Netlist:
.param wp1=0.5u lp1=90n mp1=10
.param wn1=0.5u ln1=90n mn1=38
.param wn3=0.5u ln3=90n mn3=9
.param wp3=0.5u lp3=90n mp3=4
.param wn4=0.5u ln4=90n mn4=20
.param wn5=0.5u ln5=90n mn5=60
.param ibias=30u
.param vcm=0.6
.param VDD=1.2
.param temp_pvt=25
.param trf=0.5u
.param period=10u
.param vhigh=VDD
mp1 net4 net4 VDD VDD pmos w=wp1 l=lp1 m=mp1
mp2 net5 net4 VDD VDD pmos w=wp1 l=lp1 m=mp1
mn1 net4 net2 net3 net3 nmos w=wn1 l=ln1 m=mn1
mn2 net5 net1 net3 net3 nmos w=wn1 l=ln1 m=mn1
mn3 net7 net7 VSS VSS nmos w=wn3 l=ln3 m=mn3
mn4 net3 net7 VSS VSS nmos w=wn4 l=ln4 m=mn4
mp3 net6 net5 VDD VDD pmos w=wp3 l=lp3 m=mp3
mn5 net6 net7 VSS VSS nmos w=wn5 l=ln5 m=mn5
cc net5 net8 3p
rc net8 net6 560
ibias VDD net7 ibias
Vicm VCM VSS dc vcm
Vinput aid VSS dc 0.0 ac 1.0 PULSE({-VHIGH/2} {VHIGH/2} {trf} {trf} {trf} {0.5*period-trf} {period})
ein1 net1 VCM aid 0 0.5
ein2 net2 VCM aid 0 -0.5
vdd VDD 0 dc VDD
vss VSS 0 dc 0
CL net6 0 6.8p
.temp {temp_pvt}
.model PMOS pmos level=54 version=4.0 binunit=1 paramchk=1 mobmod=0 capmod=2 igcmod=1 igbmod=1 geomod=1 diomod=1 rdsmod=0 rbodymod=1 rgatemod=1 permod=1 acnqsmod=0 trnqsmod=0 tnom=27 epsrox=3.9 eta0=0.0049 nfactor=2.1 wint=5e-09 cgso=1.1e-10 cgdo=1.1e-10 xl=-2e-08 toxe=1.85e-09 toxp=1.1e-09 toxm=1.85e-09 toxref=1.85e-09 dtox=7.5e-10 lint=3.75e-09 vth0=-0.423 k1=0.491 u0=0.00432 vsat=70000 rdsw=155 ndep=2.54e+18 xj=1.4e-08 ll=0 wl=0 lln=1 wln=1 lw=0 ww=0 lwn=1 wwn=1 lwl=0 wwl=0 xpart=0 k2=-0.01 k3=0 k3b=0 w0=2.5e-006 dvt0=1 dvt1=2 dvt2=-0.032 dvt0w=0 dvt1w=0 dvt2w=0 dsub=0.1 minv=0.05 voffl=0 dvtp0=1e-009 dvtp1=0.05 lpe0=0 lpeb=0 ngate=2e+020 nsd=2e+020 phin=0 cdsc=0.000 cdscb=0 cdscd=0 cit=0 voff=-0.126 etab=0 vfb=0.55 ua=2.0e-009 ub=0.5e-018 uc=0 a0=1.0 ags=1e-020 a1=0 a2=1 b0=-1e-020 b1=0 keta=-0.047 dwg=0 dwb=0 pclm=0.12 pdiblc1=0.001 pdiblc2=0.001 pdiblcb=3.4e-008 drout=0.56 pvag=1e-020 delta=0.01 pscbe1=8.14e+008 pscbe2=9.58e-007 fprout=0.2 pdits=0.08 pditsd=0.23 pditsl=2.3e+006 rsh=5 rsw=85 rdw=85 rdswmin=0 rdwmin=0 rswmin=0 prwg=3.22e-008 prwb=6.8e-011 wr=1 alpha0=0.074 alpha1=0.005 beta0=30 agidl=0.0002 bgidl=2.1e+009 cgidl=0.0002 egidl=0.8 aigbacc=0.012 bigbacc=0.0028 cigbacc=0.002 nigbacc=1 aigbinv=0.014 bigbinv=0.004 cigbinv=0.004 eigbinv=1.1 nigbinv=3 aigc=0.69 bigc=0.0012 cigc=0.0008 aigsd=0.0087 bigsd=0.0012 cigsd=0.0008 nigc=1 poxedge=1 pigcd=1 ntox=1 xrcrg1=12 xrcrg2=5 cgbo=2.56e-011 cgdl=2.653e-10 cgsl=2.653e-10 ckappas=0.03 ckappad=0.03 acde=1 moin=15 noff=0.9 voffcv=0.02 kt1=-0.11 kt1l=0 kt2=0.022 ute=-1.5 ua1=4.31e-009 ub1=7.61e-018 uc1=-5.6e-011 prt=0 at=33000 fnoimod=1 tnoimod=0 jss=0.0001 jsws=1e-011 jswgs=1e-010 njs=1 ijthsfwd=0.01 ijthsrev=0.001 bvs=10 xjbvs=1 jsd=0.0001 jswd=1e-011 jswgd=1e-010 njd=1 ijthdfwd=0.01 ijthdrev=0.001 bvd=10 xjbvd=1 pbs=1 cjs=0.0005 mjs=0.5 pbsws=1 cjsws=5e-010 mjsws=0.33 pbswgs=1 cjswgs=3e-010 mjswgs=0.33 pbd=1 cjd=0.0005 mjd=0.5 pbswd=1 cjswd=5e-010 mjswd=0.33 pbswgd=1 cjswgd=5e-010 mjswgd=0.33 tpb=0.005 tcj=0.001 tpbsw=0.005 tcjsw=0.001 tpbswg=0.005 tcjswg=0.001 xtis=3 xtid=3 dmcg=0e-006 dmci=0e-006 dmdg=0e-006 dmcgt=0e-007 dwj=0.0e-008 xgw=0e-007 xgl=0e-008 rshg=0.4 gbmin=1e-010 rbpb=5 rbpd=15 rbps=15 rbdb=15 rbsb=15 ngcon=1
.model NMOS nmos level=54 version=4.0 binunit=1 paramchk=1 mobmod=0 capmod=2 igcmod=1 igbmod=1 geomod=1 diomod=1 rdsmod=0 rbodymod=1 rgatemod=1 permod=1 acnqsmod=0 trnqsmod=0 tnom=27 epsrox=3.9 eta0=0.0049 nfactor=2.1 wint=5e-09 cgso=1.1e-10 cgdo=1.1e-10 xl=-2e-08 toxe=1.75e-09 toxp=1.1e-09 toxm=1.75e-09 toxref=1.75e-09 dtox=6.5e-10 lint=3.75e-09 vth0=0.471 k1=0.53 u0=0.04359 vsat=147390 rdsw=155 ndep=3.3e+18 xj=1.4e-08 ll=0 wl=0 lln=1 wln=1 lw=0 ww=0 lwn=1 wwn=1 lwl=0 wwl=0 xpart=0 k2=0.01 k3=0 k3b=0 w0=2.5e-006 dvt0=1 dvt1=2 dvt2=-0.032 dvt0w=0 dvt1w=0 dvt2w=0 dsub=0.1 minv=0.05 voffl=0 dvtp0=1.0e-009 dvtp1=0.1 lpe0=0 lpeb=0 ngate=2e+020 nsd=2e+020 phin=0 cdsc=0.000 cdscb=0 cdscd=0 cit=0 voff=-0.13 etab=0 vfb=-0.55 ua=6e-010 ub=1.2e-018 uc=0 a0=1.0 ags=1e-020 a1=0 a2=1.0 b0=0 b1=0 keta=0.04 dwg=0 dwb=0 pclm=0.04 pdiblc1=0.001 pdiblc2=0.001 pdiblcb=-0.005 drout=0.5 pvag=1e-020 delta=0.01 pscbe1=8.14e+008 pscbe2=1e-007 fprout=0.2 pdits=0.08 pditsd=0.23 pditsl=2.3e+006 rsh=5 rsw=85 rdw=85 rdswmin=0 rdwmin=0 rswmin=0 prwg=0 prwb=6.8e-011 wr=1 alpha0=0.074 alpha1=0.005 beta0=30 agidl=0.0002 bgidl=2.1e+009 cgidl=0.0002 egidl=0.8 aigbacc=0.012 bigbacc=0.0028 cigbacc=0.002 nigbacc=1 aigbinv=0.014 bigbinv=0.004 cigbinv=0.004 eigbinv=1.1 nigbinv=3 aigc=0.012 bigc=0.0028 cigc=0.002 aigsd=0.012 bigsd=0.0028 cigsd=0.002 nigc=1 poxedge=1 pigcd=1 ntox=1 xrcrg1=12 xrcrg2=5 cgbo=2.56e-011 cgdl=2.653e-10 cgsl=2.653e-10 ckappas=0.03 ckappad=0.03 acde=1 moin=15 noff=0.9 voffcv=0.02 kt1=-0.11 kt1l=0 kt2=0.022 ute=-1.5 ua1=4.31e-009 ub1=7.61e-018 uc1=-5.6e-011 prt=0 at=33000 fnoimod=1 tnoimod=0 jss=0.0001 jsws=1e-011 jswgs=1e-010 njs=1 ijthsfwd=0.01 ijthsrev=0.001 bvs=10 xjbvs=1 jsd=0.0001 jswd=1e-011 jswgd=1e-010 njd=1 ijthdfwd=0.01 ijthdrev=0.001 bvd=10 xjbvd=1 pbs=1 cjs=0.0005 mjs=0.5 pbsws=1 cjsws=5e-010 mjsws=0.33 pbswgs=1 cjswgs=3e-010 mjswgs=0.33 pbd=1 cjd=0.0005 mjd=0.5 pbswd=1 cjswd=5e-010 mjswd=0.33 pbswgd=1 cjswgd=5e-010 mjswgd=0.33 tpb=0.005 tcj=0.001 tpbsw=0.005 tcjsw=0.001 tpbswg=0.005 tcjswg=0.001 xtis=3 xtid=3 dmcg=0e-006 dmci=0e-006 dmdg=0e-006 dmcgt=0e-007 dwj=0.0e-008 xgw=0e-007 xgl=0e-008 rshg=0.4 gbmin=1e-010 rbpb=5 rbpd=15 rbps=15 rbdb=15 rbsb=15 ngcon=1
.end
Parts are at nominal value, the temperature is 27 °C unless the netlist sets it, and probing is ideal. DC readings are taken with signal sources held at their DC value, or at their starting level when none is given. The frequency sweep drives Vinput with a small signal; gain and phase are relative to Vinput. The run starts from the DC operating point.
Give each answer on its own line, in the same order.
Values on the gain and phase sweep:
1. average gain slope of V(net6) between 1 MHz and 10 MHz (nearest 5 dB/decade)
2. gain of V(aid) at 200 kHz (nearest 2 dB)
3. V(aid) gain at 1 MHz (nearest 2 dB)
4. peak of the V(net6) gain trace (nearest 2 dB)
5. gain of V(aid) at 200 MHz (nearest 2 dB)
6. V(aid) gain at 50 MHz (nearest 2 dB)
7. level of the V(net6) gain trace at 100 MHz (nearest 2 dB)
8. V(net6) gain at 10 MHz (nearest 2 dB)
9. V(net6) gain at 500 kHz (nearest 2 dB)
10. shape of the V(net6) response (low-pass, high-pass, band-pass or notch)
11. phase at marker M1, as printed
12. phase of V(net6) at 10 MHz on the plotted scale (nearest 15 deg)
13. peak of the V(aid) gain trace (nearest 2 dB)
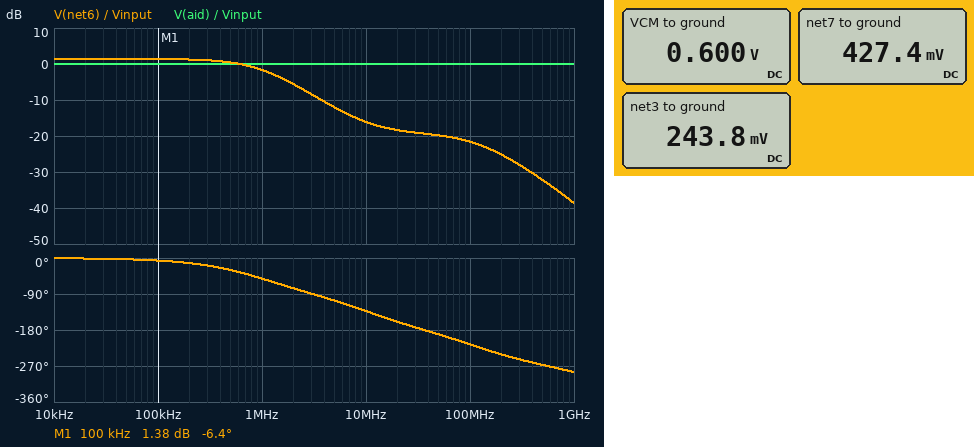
-15 dB/decade
0 dB
0 dB
2 dB
0 dB
0 dB
-22 dB
-16 dB
0 dB
low-pass
-6.4 deg
-135 deg
0 dB
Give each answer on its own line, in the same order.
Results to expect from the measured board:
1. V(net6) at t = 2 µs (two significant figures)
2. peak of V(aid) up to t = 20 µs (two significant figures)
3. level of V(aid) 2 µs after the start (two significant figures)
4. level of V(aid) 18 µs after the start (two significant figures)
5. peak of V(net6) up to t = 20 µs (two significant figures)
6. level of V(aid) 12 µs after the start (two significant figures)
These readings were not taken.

820 mV
600 mV
600 mV
-600 mV
820 mV
600 mV
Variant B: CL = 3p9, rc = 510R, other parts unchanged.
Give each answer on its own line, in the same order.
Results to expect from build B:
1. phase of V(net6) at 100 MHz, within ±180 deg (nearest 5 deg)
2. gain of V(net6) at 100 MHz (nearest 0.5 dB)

160 deg
-20.0 dB
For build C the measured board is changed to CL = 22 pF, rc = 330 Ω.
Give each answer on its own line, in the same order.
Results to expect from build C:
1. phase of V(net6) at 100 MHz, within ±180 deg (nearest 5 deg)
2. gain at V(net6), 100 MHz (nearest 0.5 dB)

115 deg
-28.0 dB
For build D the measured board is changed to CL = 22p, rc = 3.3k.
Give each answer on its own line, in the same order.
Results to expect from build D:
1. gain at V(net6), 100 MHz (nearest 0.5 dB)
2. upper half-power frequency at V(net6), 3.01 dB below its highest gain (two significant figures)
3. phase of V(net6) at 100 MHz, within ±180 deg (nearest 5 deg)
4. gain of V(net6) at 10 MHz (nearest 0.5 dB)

-35.5 dB
930 kHz
120 deg
-19.0 dB
